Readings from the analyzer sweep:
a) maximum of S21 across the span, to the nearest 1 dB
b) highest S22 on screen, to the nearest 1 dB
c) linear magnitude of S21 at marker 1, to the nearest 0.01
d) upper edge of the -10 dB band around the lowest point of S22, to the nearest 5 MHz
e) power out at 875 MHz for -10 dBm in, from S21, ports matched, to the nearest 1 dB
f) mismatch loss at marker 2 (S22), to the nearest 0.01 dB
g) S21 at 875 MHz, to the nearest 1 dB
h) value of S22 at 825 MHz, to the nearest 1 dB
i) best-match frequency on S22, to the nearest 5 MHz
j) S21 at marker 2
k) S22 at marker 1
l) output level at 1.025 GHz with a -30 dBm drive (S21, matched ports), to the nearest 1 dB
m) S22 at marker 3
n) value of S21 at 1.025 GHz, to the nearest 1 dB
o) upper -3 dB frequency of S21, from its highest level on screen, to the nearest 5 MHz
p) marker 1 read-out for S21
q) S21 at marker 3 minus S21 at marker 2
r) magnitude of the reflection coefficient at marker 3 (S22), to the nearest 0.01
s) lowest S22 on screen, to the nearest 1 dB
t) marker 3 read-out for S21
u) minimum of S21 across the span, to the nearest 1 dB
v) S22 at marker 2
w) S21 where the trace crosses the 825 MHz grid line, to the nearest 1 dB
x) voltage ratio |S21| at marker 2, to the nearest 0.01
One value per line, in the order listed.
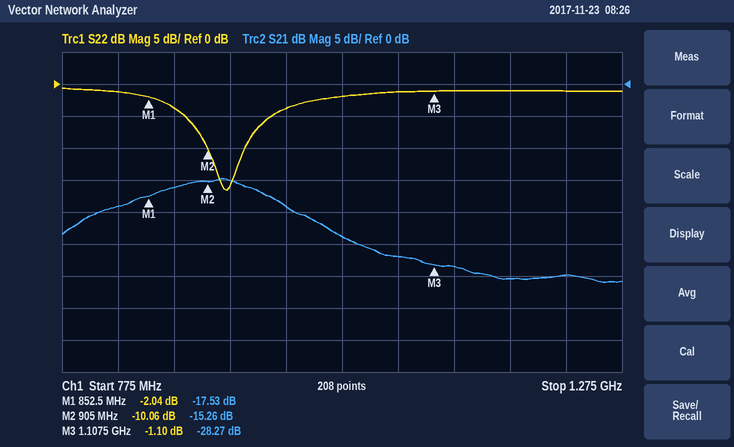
-15 dB
-1 dB
0.13
940 MHz
-26 dBm
0.45 dB
-16 dB
-1 dB
920 MHz
-15.26 dB
-2.04 dB
-54 dBm
-1.10 dB
-24 dB
965 MHz
-17.53 dB
-13.01 dB
0.88
-17 dB
-28.27 dB
-31 dB
-10.06 dB
-19 dB
0.17
